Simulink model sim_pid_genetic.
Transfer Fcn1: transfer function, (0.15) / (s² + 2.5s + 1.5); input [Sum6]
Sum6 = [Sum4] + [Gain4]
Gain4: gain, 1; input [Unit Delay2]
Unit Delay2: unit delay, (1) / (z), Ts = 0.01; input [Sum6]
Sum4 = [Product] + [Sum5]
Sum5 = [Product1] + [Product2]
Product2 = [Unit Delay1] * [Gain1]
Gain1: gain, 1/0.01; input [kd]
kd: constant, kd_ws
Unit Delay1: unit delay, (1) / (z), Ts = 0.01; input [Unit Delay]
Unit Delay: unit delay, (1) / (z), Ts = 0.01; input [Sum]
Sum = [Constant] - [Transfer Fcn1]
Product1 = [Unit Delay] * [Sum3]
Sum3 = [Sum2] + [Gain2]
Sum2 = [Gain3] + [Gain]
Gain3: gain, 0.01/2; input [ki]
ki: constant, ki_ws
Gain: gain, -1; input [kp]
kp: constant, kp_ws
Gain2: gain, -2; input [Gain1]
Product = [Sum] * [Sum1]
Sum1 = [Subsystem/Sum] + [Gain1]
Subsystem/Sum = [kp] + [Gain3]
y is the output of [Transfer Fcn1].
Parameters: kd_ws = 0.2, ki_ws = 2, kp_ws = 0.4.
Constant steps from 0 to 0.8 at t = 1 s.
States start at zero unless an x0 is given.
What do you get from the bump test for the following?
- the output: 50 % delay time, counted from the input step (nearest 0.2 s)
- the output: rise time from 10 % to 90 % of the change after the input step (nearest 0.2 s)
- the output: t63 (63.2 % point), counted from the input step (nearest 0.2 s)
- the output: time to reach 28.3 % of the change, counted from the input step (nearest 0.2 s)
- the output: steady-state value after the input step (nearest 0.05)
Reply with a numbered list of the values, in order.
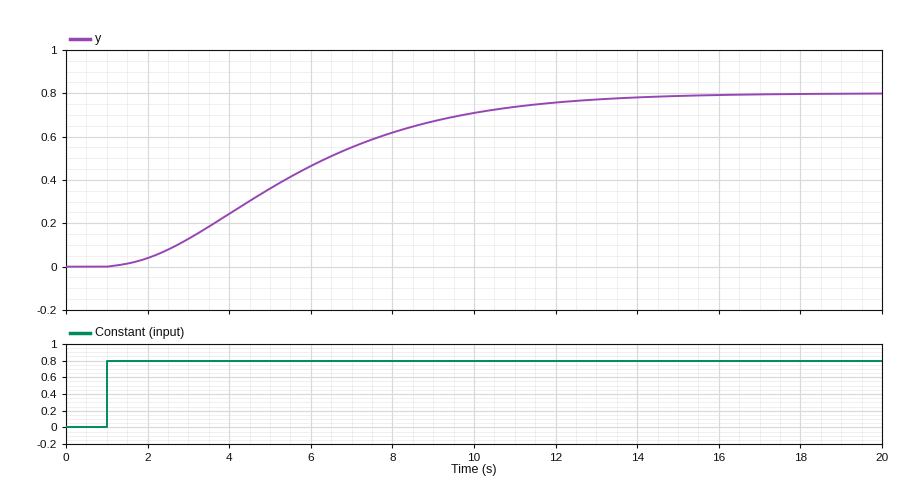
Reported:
1. 4.4 s
2. 7.8 s
3. 5.4 s
4. 2.8 s
5. 0.80
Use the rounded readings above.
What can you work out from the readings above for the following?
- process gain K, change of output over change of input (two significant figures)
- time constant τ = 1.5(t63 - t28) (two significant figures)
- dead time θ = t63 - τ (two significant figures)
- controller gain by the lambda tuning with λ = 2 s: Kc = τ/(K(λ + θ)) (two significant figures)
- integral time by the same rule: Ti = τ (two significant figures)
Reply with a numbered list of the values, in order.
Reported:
1. 1.0
2. 3.9 s
3. 1.5 s
4. 1.1
5. 3.9 s
